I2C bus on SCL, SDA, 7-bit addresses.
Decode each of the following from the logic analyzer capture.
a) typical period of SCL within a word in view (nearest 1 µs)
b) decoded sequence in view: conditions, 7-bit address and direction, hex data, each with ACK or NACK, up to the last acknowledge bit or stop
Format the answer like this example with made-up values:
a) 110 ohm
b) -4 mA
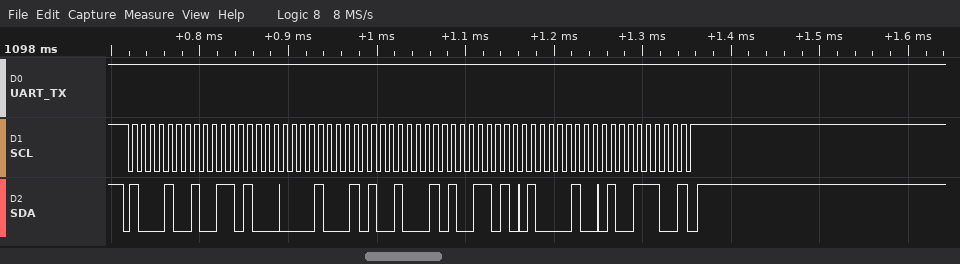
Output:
a) 10 µs
b) start, address 44 read ACK, 68 ACK, 11 ACK, 91 ACK, 9A ACK, 84 ACK, 9C NACK, stop
